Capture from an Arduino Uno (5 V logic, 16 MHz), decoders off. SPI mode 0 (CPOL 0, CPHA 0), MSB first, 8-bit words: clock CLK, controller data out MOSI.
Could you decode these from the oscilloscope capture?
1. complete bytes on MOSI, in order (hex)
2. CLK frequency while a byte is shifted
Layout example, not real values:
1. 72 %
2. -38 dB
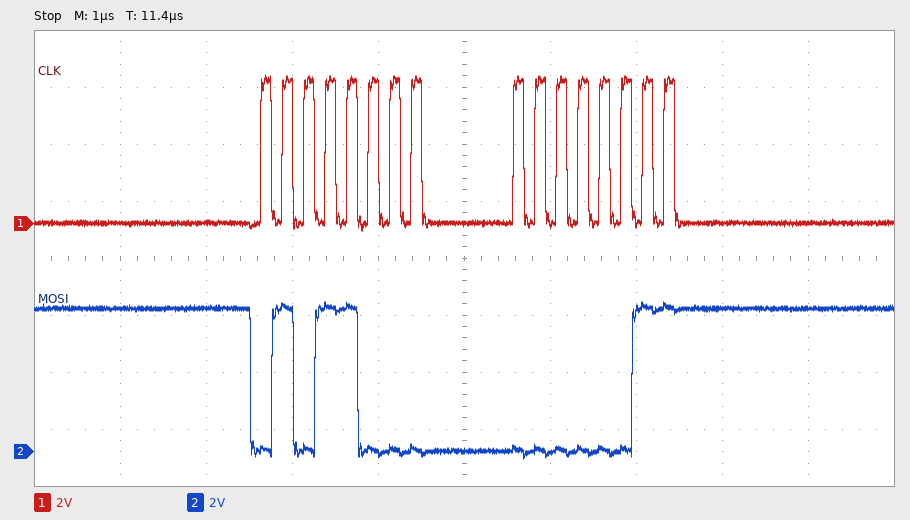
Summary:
1. 58 03
2. 4 MHz
